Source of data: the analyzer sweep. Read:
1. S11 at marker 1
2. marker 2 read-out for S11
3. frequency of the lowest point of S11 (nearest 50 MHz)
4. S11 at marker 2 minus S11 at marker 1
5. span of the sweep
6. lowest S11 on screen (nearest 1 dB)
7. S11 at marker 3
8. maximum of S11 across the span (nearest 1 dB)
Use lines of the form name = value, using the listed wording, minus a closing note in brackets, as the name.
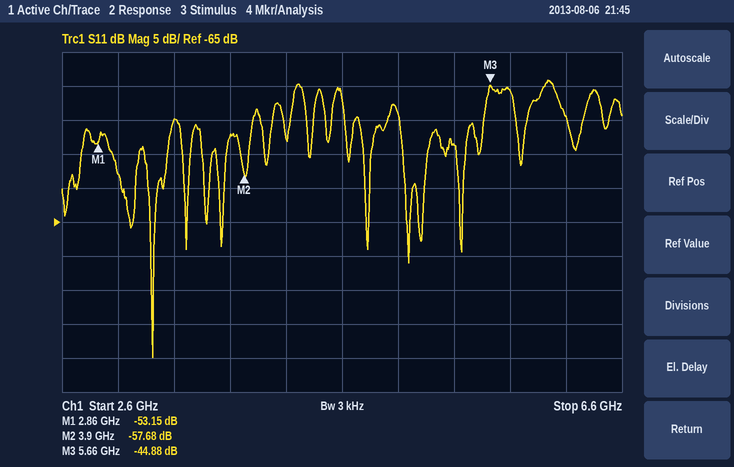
S11 at marker 1 = -53.15 dB
marker 2 read-out for S11 = -57.68 dB
frequency of the lowest point of S11 = 3.25 GHz
S11 at marker 2 minus S11 at marker 1 = -4.53 dB
span of the sweep = 4 GHz
lowest S11 on screen = -85 dB
S11 at marker 3 = -44.88 dB
maximum of S11 across the span = -44 dB
